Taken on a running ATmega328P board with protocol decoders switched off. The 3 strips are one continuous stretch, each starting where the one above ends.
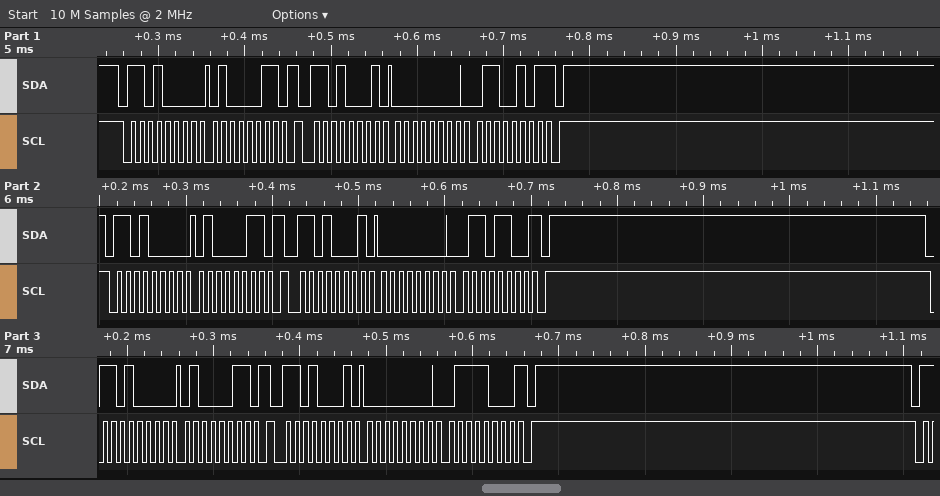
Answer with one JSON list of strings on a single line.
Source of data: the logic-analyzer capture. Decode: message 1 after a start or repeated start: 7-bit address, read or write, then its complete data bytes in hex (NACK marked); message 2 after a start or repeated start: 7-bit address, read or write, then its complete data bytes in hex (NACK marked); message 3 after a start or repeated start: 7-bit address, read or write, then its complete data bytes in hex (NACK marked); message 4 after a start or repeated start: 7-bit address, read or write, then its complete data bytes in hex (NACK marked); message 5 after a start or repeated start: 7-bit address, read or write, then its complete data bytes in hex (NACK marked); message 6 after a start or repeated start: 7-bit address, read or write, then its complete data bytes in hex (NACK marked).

["0x68 write: 43", "0x68 read: 00 65 NACK", "0x68 write: 43", "0x68 read: 00 6C NACK", "0x68 write: 43", "0x68 read: 00 78 NACK"]
